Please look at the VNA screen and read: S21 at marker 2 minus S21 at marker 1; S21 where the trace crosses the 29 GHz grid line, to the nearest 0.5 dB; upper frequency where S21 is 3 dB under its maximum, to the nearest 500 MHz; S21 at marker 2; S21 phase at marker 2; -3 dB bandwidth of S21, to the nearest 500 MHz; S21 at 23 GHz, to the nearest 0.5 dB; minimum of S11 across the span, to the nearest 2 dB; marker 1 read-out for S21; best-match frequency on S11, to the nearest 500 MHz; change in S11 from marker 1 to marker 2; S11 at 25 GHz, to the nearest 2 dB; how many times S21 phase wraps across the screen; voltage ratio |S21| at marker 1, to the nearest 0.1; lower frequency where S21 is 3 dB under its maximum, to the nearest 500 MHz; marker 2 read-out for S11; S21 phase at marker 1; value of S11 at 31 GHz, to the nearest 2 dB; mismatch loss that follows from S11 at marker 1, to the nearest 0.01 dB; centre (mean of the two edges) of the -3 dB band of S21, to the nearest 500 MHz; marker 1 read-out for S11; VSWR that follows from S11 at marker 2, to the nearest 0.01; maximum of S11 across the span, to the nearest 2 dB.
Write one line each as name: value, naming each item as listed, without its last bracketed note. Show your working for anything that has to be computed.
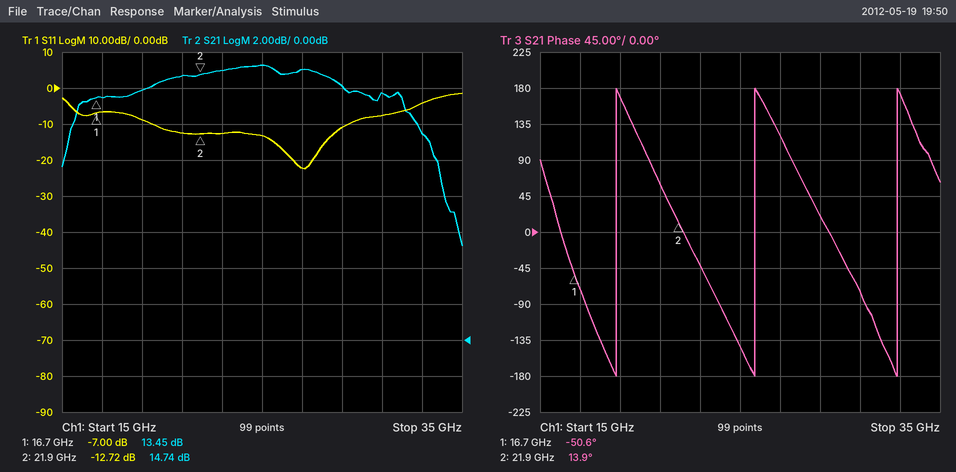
S21 at marker 2 minus S21 at marker 1: 14.74 − (13.45) = 1.29 dB
S21 where the trace crosses the 29 GHz grid line, to the nearest 0.5 dB: 14.0 dB
upper frequency where S21 is 3 dB under its maximum, to the nearest 500 MHz: 32.5 GHz
S21 at marker 2: 14.74 dB
S21 phase at marker 2: 13.9°
-3 dB bandwidth of S21, to the nearest 500 MHz: 32.5 GHz − 15.5 GHz = 17.0 GHz
S21 at 23 GHz, to the nearest 0.5 dB: 15.0 dB
minimum of S11 across the span, to the nearest 2 dB: -22 dB
marker 1 read-out for S21: 13.45 dB
best-match frequency on S11, to the nearest 500 MHz: 27.0 GHz
change in S11 from marker 1 to marker 2: -12.72 − (-7) = -5.72 dB
S11 at 25 GHz, to the nearest 2 dB: -14 dB
how many times S21 phase wraps across the screen: 3
voltage ratio |S21| at marker 1, to the nearest 0.1: 10^(13.45/20) ≈ 4.7
lower frequency where S21 is 3 dB under its maximum, to the nearest 500 MHz: 15.5 GHz
marker 2 read-out for S11: -12.72 dB
S21 phase at marker 1: -50.6°
value of S11 at 31 GHz, to the nearest 2 dB: -8 dB
mismatch loss that follows from S11 at marker 1, to the nearest 0.01 dB: −10 log10(1 − 10^(-7/10)) ≈ 0.97 dB
centre (mean of the two edges) of the -3 dB band of S21, to the nearest 500 MHz: 24.0 GHz
marker 1 read-out for S11: -7.00 dB
VSWR that follows from S11 at marker 2, to the nearest 0.01: (1 + 0.2312)/(1 − 0.2312) ≈ 1.60
maximum of S11 across the span, to the nearest 2 dB: -2 dB
